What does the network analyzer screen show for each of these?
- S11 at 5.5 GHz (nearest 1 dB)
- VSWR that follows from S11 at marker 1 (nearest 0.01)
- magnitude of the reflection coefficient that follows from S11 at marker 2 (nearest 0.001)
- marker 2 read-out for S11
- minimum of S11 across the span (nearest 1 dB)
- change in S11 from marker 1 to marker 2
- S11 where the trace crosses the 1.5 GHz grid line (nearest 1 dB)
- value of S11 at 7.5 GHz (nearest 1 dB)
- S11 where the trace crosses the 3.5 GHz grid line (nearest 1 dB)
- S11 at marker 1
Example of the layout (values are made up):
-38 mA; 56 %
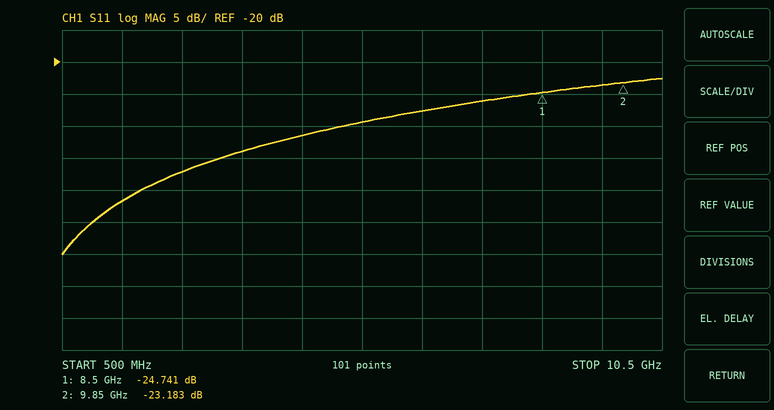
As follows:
-29 dB; 1.12; 0.069; -23.183 dB; -50 dB; 1.558 dB; -42 dB; -26 dB; -34 dB; -24.741 dB
